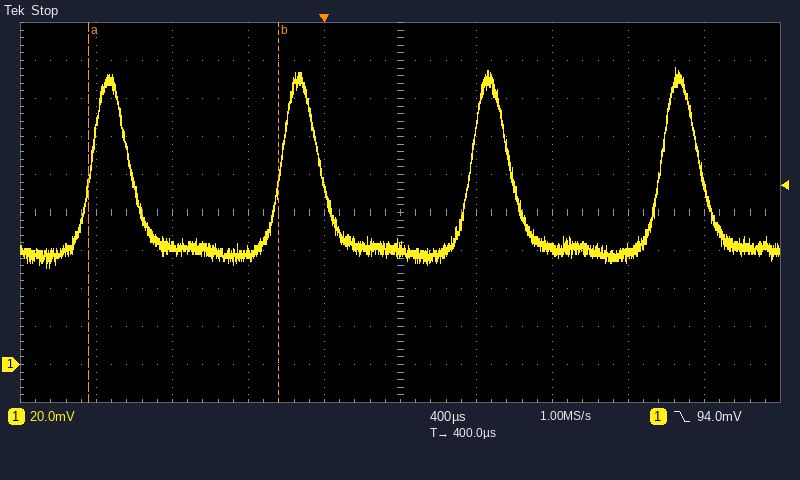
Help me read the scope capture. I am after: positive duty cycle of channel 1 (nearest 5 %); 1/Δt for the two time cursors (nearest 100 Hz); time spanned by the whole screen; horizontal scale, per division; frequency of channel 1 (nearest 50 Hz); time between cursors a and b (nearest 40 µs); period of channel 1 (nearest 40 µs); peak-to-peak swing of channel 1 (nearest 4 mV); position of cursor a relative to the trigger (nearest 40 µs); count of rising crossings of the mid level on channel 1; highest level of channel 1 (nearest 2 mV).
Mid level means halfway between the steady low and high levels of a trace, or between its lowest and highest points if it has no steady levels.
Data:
20 %
1.0 kHz
4 ms
400 µs
1.00 kHz
1.00 ms
1.00 ms
104 mV
-1.24 ms
4
156 mV
